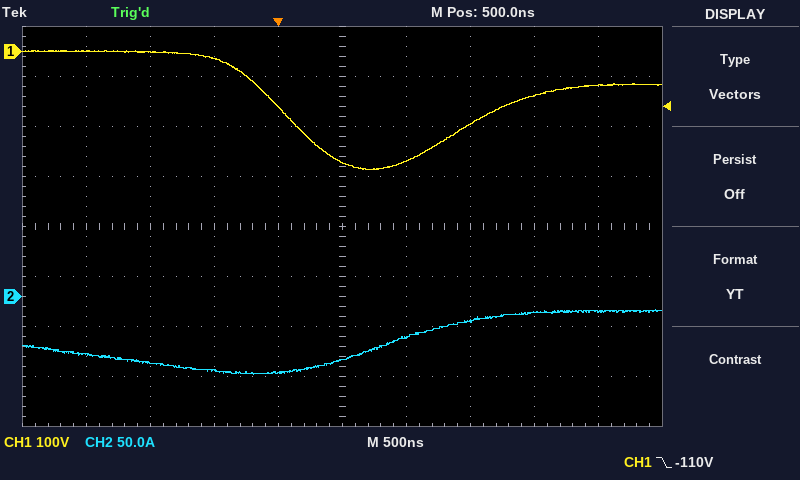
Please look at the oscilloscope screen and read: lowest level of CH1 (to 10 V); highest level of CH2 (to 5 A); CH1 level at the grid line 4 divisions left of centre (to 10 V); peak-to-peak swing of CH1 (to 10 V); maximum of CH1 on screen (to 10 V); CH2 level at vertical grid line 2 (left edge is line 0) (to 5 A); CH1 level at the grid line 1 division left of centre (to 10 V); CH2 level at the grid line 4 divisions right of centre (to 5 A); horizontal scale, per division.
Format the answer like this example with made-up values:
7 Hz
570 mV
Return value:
-240 V
-15 A
0 V
240 V
0 V
-65 A
-110 V
-15 A
500 ns
